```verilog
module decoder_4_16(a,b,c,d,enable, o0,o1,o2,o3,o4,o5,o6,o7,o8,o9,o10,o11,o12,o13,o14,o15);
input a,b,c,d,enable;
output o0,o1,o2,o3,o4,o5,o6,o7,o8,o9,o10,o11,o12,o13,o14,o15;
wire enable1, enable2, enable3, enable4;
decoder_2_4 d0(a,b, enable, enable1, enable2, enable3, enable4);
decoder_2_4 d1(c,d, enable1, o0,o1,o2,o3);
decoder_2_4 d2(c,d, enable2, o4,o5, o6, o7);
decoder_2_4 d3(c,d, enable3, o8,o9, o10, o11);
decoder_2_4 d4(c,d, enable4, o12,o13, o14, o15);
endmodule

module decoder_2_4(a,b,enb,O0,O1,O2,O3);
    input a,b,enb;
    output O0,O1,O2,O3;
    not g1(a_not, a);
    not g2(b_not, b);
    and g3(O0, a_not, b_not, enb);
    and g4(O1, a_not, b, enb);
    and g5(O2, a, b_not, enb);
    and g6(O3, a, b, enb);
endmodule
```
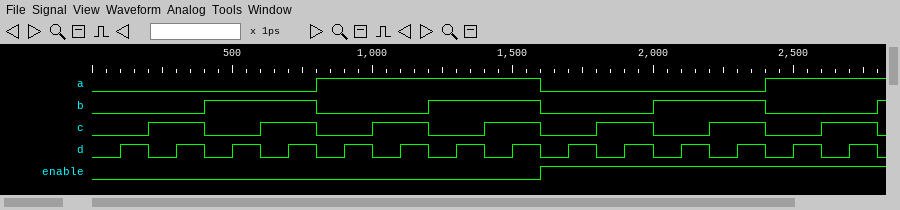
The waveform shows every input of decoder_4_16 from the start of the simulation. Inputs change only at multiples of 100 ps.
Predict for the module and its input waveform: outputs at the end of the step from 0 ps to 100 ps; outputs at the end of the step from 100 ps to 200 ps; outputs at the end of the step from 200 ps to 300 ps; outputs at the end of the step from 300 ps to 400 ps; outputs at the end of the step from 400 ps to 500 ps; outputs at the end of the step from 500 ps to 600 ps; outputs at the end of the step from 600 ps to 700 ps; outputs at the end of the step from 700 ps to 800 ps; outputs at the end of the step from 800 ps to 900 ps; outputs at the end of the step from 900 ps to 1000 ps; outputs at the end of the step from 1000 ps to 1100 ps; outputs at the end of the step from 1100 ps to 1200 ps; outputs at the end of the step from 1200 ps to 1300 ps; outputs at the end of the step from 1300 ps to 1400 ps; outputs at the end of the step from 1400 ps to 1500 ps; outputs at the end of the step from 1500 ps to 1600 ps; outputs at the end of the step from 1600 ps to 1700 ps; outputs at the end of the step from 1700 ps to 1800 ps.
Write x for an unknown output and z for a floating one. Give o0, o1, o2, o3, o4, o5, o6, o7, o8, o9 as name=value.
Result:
o0=0, o1=0, o2=0, o3=0, o4=0, o5=0, o6=0, o7=0, o8=0, o9=0
o0=0, o1=0, o2=0, o3=0, o4=0, o5=0, o6=0, o7=0, o8=0, o9=0
o0=0, o1=0, o2=0, o3=0, o4=0, o5=0, o6=0, o7=0, o8=0, o9=0
o0=0, o1=0, o2=0, o3=0, o4=0, o5=0, o6=0, o7=0, o8=0, o9=0
o0=0, o1=0, o2=0, o3=0, o4=0, o5=0, o6=0, o7=0, o8=0, o9=0
o0=0, o1=0, o2=0, o3=0, o4=0, o5=0, o6=0, o7=0, o8=0, o9=0
o0=0, o1=0, o2=0, o3=0, o4=0, o5=0, o6=0, o7=0, o8=0, o9=0
o0=0, o1=0, o2=0, o3=0, o4=0, o5=0, o6=0, o7=0, o8=0, o9=0
o0=0, o1=0, o2=0, o3=0, o4=0, o5=0, o6=0, o7=0, o8=0, o9=0
o0=0, o1=0, o2=0, o3=0, o4=0, o5=0, o6=0, o7=0, o8=0, o9=0
o0=0, o1=0, o2=0, o3=0, o4=0, o5=0, o6=0, o7=0, o8=0, o9=0
o0=0, o1=0, o2=0, o3=0, o4=0, o5=0, o6=0, o7=0, o8=0, o9=0
o0=0, o1=0, o2=0, o3=0, o4=0, o5=0, o6=0, o7=0, o8=0, o9=0
o0=0, o1=0, o2=0, o3=0, o4=0, o5=0, o6=0, o7=0, o8=0, o9=0
o0=0, o1=0, o2=0, o3=0, o4=0, o5=0, o6=0, o7=0, o8=0, o9=0
o0=0, o1=0, o2=0, o3=0, o4=0, o5=0, o6=0, o7=0, o8=0, o9=0
o0=1, o1=0, o2=0, o3=0, o4=0, o5=0, o6=0, o7=0, o8=0, o9=0
o0=0, o1=1, o2=0, o3=0, o4=0, o5=0, o6=0, o7=0, o8=0, o9=0
